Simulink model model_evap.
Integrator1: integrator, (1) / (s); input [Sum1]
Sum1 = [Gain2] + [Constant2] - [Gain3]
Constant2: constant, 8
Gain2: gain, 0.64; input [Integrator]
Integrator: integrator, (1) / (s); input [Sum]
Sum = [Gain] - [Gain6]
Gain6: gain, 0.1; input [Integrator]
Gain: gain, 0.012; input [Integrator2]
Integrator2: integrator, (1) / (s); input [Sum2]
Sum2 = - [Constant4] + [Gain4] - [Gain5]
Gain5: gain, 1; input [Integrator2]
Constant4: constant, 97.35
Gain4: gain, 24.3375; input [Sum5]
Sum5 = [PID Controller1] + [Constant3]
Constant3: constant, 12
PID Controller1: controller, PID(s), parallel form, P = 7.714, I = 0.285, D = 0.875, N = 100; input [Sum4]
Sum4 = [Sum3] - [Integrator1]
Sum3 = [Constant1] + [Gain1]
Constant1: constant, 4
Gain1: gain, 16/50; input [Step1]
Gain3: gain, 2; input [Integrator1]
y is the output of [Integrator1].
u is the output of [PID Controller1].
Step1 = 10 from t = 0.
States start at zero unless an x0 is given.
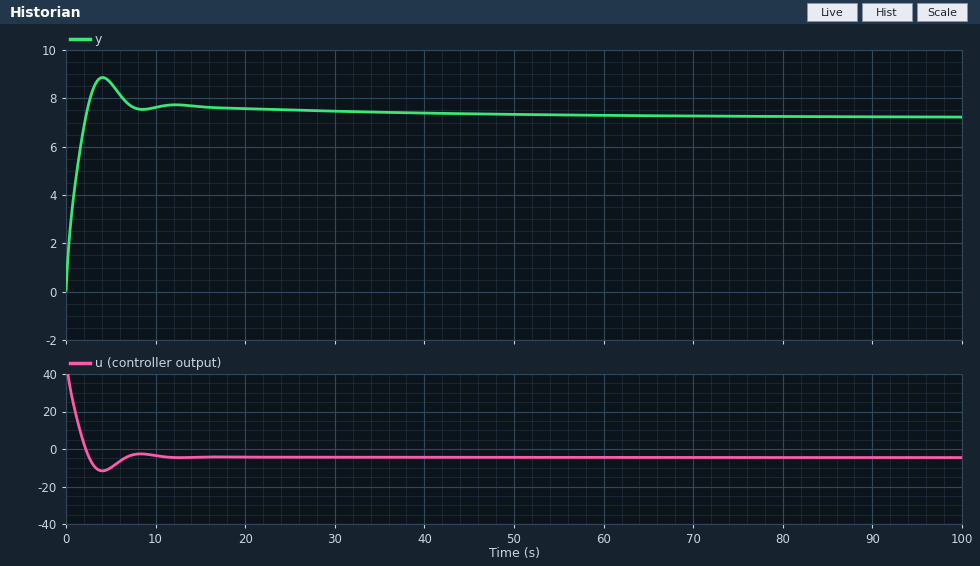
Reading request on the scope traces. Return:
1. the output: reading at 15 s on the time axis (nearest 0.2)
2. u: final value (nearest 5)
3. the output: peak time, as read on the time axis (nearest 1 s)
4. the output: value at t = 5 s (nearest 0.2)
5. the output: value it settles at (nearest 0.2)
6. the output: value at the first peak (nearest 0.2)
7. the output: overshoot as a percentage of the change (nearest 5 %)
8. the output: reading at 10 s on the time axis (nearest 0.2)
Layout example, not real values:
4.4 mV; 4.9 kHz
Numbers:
7.6; -5; 4 s; 8.6; 7.2; 8.8; 25 %; 7.6
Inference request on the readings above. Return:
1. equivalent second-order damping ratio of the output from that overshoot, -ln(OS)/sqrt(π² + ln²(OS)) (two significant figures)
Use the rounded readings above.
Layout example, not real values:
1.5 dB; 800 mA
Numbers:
0.40
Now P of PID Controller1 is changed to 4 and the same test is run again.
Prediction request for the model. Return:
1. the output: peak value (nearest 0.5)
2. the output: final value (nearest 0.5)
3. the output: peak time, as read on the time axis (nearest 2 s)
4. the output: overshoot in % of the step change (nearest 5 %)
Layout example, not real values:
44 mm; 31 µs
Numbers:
8.5; 7.0; 6 s; 20 %
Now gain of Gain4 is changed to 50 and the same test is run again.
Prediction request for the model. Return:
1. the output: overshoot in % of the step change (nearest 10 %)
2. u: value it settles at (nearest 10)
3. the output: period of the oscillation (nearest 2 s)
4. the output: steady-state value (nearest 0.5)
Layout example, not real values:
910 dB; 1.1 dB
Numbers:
50 %; -10; 6 s; 7.0
